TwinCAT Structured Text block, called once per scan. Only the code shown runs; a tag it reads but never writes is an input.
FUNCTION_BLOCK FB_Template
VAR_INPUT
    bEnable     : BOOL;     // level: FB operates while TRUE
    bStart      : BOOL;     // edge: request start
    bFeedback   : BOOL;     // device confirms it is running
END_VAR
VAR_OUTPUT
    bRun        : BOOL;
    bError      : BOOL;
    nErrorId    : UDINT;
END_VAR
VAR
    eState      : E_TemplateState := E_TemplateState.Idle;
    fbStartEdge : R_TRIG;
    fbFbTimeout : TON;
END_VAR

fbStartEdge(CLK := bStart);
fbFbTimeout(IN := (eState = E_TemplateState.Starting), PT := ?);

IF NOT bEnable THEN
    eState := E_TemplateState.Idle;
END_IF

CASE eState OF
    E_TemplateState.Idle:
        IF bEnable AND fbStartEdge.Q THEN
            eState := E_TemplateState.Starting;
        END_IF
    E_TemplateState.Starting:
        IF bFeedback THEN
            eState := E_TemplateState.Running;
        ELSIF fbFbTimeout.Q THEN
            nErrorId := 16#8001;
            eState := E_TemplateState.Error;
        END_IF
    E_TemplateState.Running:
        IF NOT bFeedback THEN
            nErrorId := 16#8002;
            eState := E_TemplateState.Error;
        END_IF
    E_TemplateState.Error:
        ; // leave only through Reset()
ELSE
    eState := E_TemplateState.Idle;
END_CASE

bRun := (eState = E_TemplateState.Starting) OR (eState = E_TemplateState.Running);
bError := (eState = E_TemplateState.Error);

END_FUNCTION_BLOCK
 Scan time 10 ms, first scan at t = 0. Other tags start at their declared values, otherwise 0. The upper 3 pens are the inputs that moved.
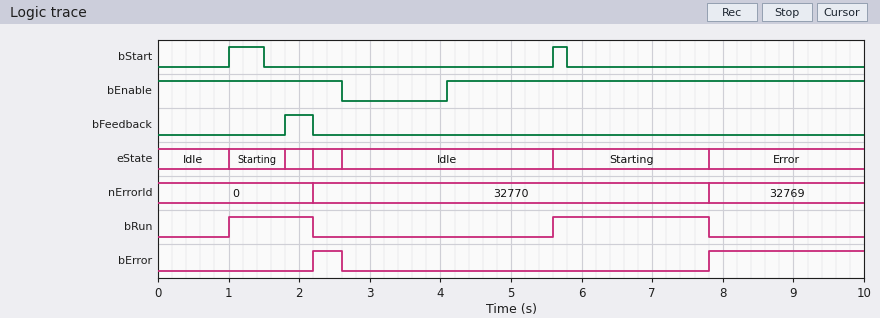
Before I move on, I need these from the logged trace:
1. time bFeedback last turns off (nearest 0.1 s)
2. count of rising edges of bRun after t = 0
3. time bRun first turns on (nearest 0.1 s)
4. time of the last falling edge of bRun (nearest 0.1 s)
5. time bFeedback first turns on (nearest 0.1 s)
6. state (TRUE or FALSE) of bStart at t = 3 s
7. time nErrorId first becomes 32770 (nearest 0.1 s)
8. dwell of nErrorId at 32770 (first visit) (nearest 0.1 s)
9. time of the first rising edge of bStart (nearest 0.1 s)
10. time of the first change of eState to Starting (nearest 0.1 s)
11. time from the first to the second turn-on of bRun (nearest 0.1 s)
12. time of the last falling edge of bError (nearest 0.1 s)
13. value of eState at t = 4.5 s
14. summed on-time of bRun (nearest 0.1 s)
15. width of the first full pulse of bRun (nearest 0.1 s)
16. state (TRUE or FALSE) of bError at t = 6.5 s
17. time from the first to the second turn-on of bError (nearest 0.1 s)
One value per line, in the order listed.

2.2 s
2
1.0 s
7.8 s
1.8 s
FALSE
2.2 s
5.6 s
1.0 s
1.0 s
4.6 s
2.6 s
Idle
3.4 s
1.2 s
FALSE
5.6 s
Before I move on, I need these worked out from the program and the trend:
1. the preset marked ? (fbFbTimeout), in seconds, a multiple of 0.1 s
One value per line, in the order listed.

2.2 s
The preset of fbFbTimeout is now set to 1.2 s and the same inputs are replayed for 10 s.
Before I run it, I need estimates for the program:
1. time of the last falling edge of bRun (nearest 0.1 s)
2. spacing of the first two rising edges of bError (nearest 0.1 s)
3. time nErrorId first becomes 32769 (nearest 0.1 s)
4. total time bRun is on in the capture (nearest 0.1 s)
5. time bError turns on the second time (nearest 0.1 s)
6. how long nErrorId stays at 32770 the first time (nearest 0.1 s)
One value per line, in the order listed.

6.8 s
4.6 s
6.8 s
2.4 s
6.8 s
4.6 s
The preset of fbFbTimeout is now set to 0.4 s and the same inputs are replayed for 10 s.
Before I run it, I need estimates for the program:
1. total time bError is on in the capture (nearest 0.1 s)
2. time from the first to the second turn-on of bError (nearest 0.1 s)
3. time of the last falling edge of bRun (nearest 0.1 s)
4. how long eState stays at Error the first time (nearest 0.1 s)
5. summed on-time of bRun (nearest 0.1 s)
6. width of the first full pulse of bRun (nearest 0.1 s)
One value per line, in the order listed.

5.2 s
4.6 s
6.0 s
1.2 s
0.8 s
0.4 s
